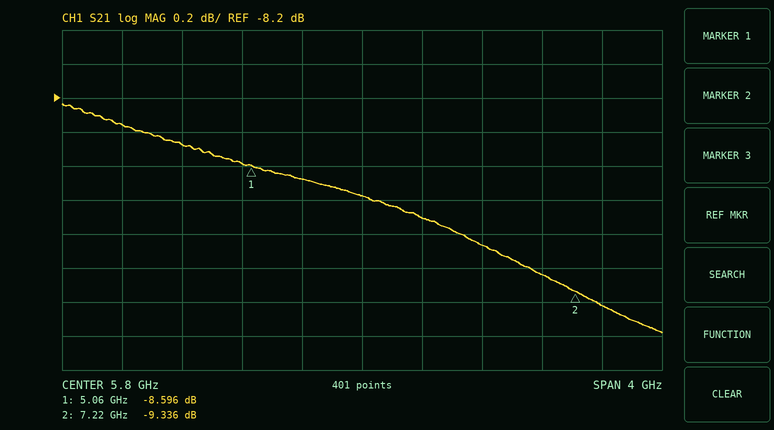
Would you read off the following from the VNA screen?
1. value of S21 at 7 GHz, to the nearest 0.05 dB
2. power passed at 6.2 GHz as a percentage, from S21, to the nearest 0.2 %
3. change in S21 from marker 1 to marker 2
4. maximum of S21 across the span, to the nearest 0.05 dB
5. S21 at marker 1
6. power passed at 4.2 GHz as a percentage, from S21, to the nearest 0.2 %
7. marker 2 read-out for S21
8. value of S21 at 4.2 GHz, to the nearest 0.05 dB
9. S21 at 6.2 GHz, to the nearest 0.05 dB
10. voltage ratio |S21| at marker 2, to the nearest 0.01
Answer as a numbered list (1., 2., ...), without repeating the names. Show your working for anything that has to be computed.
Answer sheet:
1. -9.25 dB
2. 10^(-8.9/10) ≈ 12.9 %, so 12.8 % to the nearest 0.2 %
3. -9.336 − (-8.596) = -0.740 dB
4. -8.25 dB
5. -8.596 dB
6. 10^(-8.35/10) ≈ 14.6 %
7. -9.336 dB
8. -8.35 dB
9. -8.90 dB
10. 10^(-9.336/20) ≈ 0.34
